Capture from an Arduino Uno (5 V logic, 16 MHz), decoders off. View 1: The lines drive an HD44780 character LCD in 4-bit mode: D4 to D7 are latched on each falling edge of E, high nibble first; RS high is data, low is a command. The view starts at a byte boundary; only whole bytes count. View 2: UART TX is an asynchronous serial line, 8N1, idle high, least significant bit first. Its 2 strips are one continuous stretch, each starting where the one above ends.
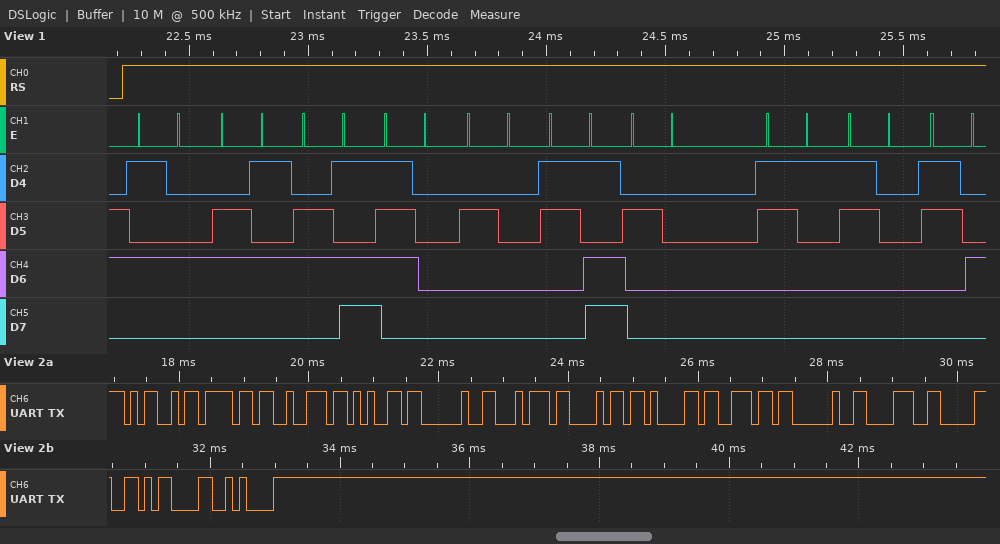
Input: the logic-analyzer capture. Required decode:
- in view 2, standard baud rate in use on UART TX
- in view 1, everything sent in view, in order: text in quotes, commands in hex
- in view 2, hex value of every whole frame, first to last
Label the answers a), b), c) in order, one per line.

a) 9600 baud
b) "Temp = 104"
c) 4D 6F 72 65 20 74 68 61 6E 20 38 30 0D 0A
